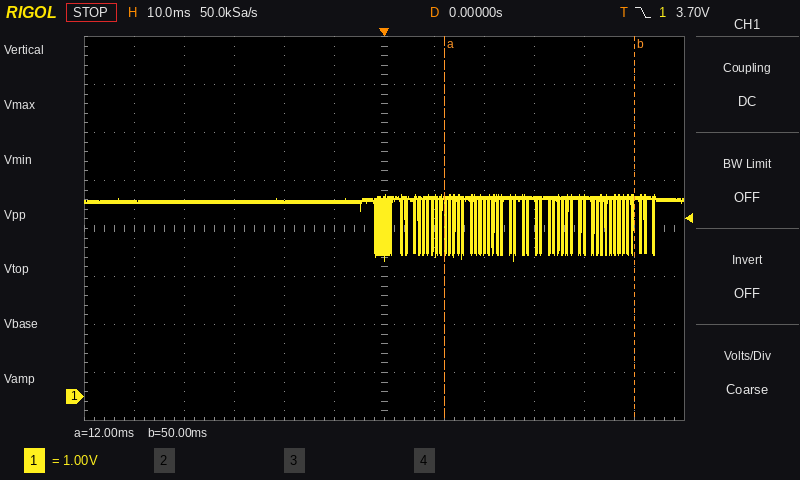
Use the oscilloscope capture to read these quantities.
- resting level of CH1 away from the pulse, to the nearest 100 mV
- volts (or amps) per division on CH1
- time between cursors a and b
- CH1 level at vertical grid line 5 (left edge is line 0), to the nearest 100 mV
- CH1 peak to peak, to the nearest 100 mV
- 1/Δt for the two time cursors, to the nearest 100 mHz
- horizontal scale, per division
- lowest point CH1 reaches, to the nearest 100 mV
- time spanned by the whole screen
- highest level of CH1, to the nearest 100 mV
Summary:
4.1 V
1 V
38 ms
4.1 V
1.4 V
26.3 Hz
10 ms
2.8 V
120 ms
4.2 V
